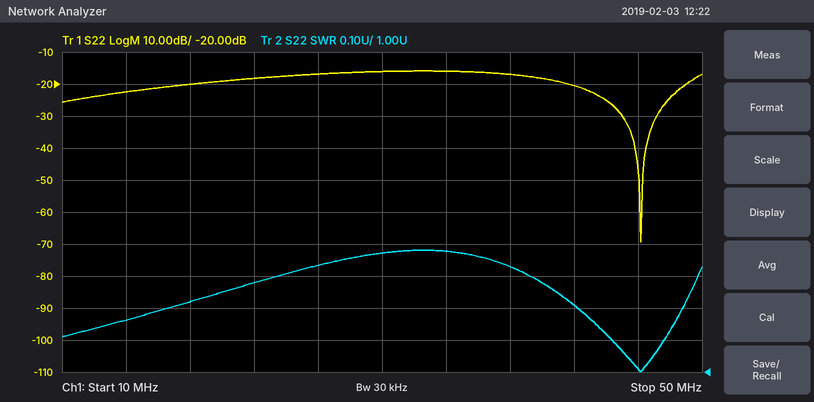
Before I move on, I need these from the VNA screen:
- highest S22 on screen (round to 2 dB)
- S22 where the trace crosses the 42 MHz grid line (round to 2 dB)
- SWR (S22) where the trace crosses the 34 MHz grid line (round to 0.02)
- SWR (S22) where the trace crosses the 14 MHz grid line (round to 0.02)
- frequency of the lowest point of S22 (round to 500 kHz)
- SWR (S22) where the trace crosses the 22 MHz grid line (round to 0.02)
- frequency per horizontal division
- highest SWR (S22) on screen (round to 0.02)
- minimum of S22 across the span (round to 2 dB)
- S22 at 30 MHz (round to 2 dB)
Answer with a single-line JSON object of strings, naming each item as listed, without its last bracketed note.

{"highest S22 on screen": "-16 dB", "S22 where the trace crosses the 42 MHz grid line": "-20 dB", "SWR (S22) where the trace crosses the 34 MHz grid line": "1.38", "SWR (S22) where the trace crosses the 14 MHz grid line": "1.16", "frequency of the lowest point of S22": "46.0 MHz", "SWR (S22) where the trace crosses the 22 MHz grid line": "1.28", "frequency per horizontal division": "4 MHz", "highest SWR (S22) on screen": "1.38", "minimum of S22 across the span": "-70 dB", "S22 at 30 MHz": "-16 dB"}
